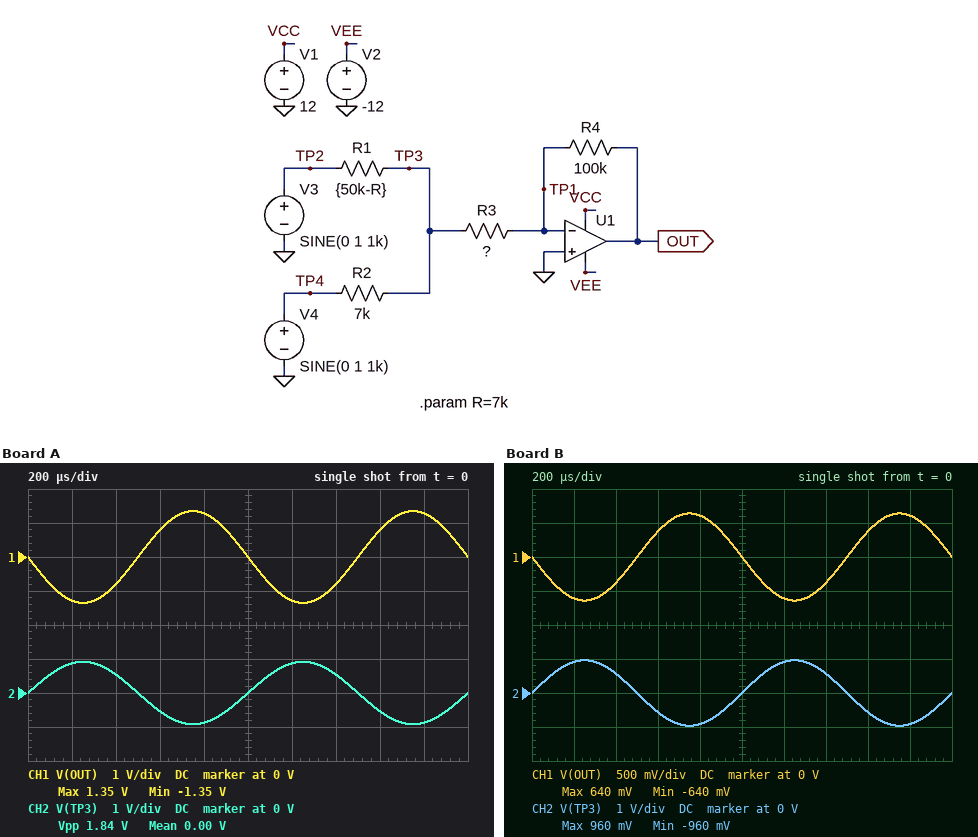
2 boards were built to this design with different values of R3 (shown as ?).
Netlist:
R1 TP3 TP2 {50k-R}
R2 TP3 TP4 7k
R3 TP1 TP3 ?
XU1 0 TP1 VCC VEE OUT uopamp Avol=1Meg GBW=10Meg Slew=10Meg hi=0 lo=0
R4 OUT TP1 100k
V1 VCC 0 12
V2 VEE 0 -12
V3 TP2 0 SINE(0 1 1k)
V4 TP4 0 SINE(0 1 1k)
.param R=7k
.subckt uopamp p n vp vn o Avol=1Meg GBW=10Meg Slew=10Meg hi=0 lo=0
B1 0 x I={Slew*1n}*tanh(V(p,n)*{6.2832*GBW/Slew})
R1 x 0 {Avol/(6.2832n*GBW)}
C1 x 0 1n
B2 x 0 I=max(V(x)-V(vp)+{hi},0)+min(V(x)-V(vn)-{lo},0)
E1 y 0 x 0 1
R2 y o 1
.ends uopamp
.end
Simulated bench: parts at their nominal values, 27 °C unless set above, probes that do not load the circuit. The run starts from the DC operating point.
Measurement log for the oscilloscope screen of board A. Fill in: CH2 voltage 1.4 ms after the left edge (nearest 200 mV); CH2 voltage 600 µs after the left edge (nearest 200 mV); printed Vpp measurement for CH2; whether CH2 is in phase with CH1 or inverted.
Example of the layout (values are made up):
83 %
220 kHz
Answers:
600 mV
-600 mV
1.84 V
inverted
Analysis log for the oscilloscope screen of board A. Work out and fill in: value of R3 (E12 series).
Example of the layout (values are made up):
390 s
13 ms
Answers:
68 kΩ
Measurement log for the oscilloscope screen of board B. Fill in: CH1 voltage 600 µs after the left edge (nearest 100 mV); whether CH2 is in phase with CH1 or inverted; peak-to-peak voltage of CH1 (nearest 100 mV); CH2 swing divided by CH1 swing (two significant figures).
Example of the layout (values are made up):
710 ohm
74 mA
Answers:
400 mV
inverted
1.3 V
1.5
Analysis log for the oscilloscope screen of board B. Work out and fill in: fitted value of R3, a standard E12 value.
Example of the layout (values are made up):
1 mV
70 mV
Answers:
150 kΩ
